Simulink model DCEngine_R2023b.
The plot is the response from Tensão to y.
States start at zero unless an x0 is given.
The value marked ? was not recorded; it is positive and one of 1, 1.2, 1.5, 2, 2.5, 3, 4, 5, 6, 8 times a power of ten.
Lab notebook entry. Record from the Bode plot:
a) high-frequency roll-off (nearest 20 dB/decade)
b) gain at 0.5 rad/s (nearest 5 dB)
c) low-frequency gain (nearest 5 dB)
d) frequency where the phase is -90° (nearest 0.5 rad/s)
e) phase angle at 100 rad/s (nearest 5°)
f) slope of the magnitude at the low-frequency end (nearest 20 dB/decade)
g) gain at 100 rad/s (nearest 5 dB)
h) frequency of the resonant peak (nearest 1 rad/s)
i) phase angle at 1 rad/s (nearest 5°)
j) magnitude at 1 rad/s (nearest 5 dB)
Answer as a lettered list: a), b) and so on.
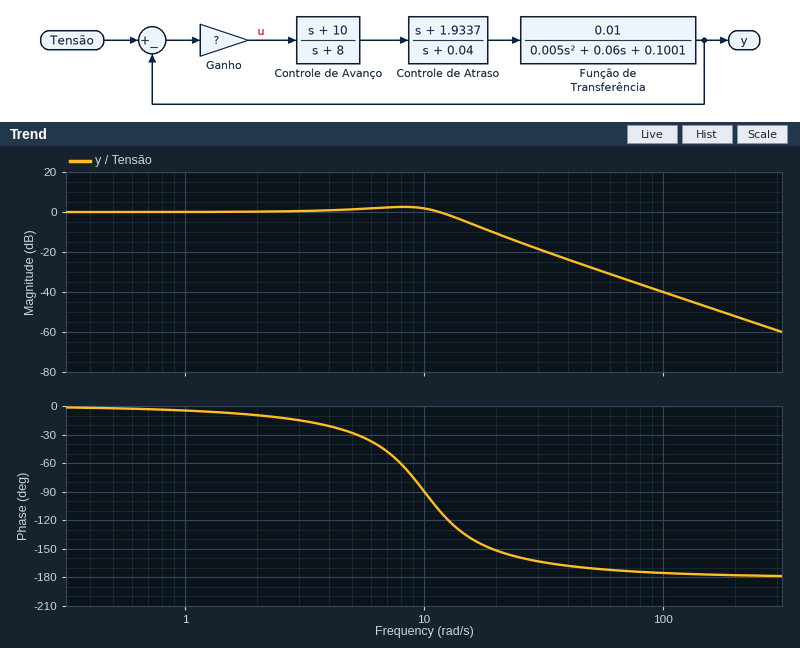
a) -40 dB/decade
b) 0 dB
c) 0 dB
d) 10.0 rad/s
e) -175°
f) 0 dB/decade
g) -40 dB
h) 8 rad/s
i) -5°
j) 0 dB
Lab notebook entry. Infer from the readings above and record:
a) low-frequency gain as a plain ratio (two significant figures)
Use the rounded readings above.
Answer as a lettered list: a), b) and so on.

a) 1.0
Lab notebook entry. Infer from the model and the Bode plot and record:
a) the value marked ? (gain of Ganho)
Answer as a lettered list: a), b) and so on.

a) 50
